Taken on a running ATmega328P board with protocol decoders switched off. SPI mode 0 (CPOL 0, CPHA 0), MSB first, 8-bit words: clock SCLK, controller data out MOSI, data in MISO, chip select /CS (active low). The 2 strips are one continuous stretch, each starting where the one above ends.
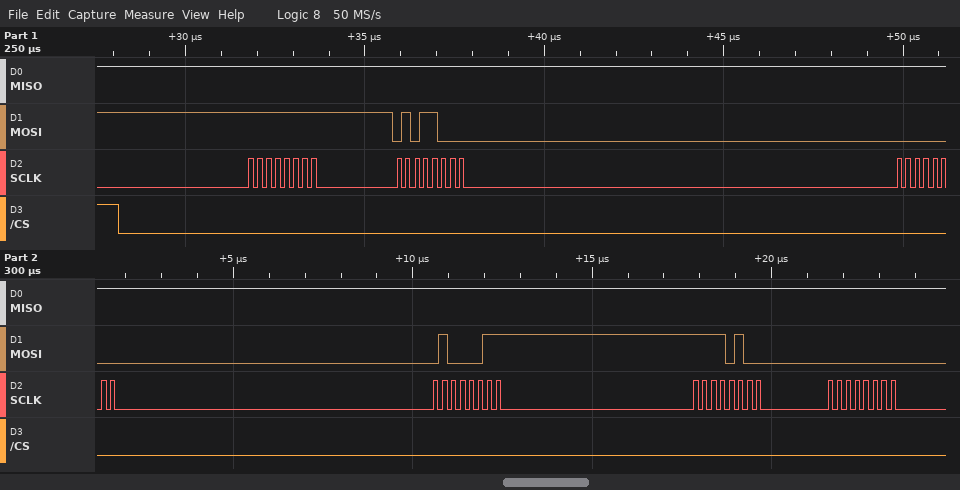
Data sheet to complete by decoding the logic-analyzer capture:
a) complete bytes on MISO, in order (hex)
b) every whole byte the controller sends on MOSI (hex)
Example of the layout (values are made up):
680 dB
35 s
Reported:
0xFF 0xFF 0xFF 0xFF 0xFF 0xFF
0xFF 0x58 0x00 0x43 0xF4 0x00
